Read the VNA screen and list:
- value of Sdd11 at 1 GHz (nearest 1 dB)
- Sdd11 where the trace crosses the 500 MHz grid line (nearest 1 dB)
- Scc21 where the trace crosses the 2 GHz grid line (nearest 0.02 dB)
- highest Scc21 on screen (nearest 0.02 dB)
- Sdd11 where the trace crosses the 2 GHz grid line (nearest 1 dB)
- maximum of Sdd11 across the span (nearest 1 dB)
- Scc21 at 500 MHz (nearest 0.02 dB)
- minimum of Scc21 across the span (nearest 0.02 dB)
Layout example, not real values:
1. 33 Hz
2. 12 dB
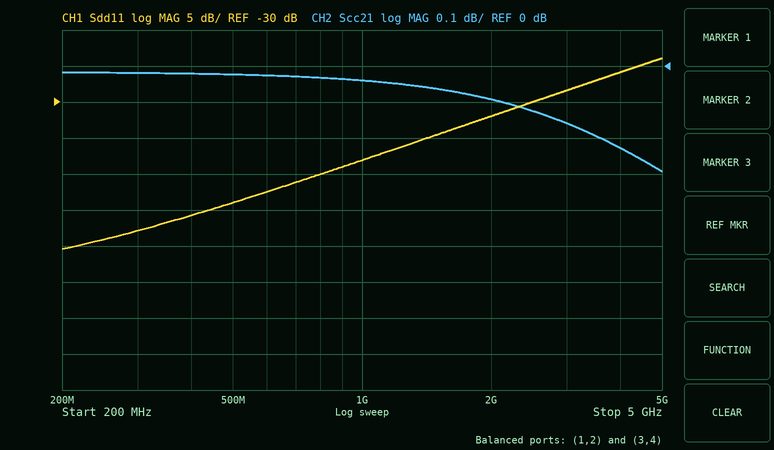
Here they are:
1. -38 dB
2. -44 dB
3. -0.10 dB
4. -0.02 dB
5. -32 dB
6. -24 dB
7. -0.02 dB
8. -0.30 dB
